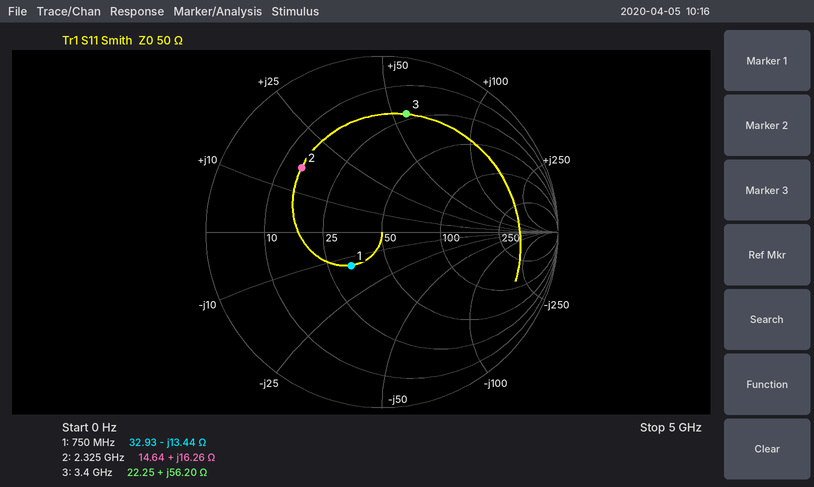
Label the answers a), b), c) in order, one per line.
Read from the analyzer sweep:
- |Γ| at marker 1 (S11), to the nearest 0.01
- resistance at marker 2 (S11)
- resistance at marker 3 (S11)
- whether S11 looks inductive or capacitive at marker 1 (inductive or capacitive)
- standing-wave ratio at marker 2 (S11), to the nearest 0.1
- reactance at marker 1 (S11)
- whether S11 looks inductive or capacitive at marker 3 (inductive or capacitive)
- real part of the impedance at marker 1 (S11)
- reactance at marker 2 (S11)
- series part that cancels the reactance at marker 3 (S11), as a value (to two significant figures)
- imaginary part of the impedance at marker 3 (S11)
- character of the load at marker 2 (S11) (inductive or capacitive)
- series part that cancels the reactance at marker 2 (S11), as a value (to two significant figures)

a) 0.26
b) 14.64 Ω
c) 22.25 Ω
d) capacitive
e) 3.8
f) -13.44 Ω
g) inductive
h) 32.93 Ω
i) +16.26 Ω
j) 830 fF
k) +56.20 Ω
l) inductive
m) 4.2 pF
